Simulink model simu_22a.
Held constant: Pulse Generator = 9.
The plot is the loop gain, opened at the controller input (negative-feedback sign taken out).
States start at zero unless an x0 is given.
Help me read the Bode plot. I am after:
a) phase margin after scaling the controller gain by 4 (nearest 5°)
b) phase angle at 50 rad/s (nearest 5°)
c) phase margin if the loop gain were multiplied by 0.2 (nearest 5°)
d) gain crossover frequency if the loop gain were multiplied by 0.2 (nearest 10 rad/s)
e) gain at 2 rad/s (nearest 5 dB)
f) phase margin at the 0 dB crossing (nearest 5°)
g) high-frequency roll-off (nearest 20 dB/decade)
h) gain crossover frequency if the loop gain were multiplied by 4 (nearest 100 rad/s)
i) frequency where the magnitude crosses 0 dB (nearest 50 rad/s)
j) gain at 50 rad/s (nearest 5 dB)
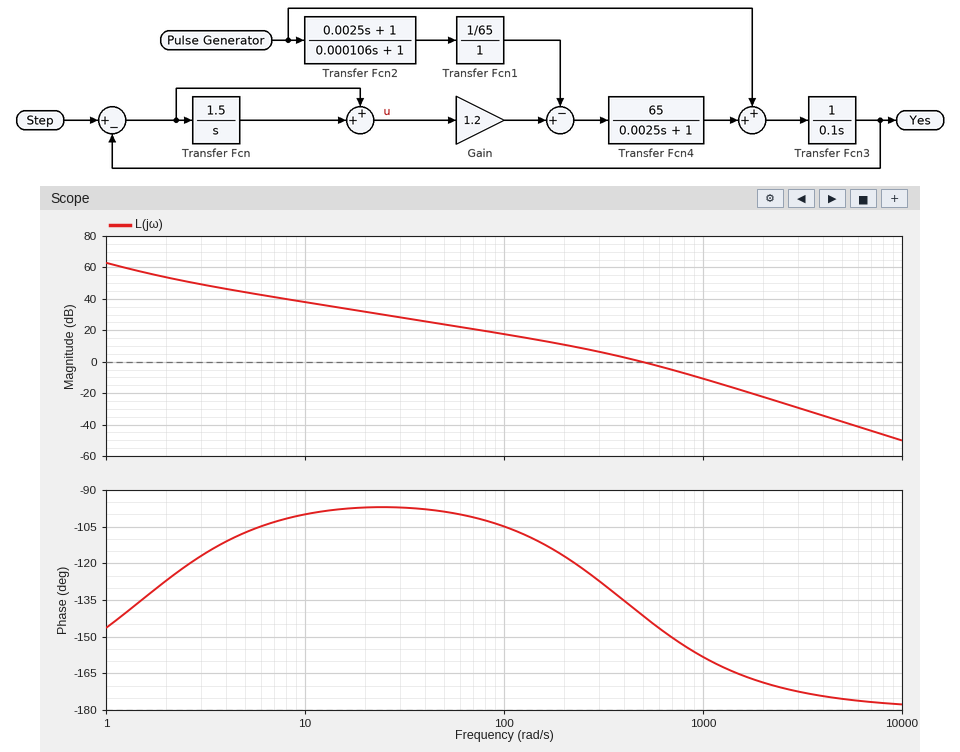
20°
-100°
70°
150 rad/s
55 dB
40°
-40 dB/decade
1100 rad/s
500 rad/s
25 dB
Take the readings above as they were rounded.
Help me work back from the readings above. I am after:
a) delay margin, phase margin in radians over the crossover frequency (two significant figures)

0.0014 s
